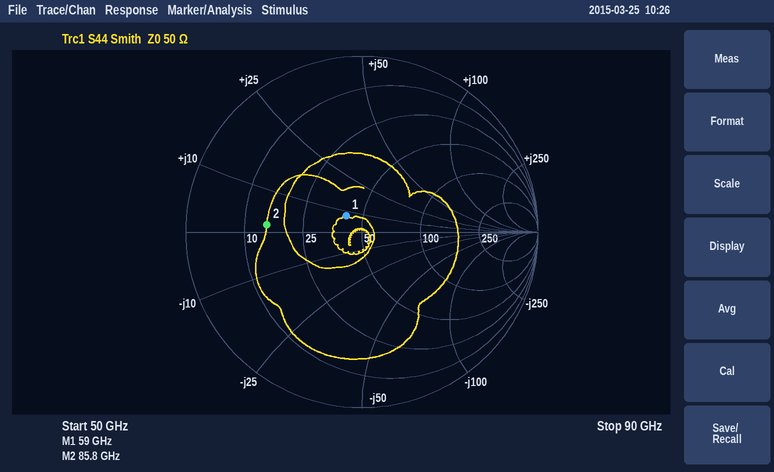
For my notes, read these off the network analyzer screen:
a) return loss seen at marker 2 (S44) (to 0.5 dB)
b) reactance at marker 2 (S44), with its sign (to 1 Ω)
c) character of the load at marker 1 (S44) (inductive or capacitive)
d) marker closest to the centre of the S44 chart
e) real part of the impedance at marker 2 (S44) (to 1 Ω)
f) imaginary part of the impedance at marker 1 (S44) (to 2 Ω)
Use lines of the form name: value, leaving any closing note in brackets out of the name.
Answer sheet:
return loss seen at marker 2 (S44): 5.5 dB
reactance at marker 2 (S44), with its sign: +2 Ω
character of the load at marker 1 (S44): inductive
marker closest to the centre of the S44 chart: marker 1
real part of the impedance at marker 2 (S44): 15 Ω
imaginary part of the impedance at marker 1 (S44): +8 Ω
